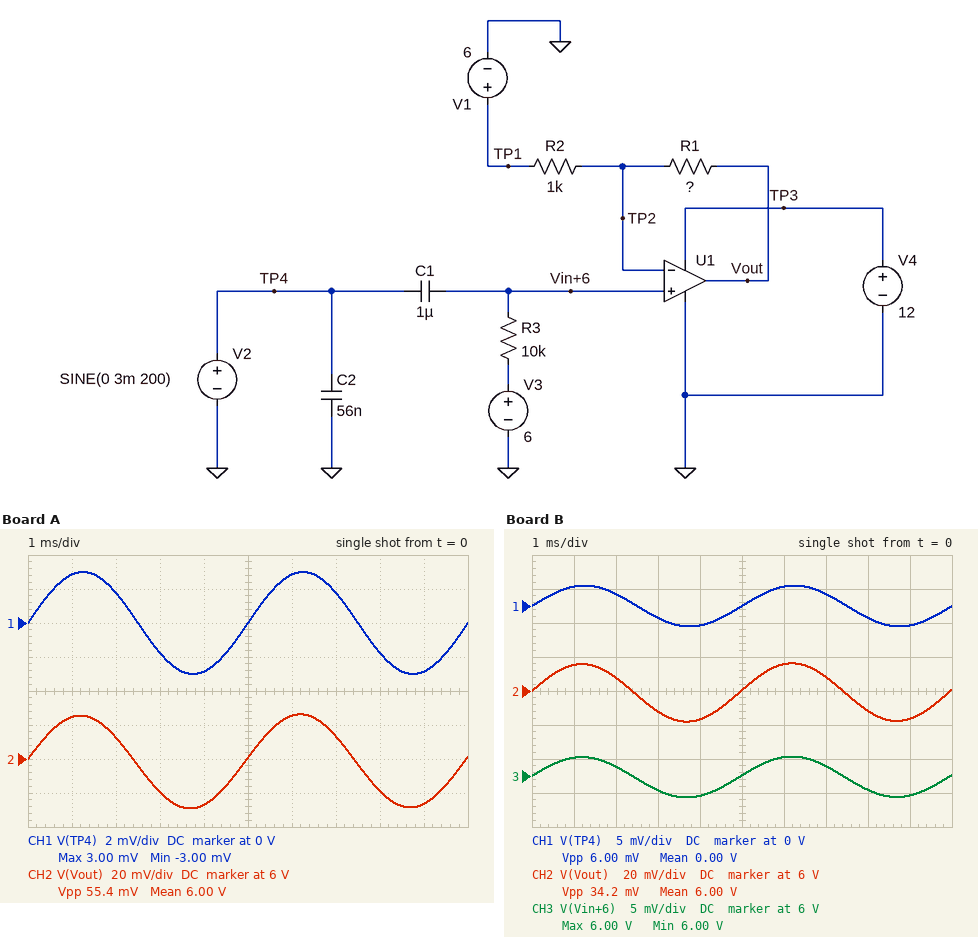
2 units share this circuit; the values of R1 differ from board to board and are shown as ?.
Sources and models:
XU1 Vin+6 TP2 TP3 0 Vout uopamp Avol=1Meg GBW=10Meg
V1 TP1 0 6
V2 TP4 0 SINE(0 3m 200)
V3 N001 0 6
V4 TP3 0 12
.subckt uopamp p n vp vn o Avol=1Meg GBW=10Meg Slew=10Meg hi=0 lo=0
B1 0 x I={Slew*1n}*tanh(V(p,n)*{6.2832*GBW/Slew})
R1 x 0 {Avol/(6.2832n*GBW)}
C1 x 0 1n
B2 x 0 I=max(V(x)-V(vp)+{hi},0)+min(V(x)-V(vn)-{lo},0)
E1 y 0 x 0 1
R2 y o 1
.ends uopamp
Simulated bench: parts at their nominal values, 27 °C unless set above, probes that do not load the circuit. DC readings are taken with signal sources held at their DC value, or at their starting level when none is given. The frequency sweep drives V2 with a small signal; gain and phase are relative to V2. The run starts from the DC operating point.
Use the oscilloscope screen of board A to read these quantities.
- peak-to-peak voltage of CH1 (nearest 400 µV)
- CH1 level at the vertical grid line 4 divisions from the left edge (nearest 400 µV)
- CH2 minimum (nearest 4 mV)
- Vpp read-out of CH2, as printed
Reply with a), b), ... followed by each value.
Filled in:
a) 6.0 mV
b) -2.8 mV
c) 5.972 V
d) 55.4 mV
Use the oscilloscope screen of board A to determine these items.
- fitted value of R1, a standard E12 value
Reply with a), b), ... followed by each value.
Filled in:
a) 8.2 kΩ
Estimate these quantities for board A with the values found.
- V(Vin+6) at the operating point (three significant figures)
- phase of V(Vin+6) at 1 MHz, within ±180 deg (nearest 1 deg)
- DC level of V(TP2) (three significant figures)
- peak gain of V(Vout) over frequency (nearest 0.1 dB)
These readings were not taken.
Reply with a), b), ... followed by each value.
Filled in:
a) 6.00 V
b) 0 deg
c) 6.00 V
d) 19.3 dB
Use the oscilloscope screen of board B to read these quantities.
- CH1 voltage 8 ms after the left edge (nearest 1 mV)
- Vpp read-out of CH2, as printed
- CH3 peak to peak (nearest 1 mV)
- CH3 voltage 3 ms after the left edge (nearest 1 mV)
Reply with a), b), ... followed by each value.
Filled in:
a) -2 mV
b) 34.2 mV
c) 6 mV
d) 5.998 V
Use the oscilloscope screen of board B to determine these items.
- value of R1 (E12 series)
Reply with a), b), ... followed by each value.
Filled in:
a) 4.7 kΩ
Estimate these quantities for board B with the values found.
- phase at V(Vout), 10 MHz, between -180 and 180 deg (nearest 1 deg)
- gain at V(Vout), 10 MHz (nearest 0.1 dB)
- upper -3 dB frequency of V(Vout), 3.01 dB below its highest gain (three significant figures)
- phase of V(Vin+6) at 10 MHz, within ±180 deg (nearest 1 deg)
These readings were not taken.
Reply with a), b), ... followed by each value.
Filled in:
a) -80 deg
b) -0.1 dB
c) 1.75 MHz
d) 0 deg
